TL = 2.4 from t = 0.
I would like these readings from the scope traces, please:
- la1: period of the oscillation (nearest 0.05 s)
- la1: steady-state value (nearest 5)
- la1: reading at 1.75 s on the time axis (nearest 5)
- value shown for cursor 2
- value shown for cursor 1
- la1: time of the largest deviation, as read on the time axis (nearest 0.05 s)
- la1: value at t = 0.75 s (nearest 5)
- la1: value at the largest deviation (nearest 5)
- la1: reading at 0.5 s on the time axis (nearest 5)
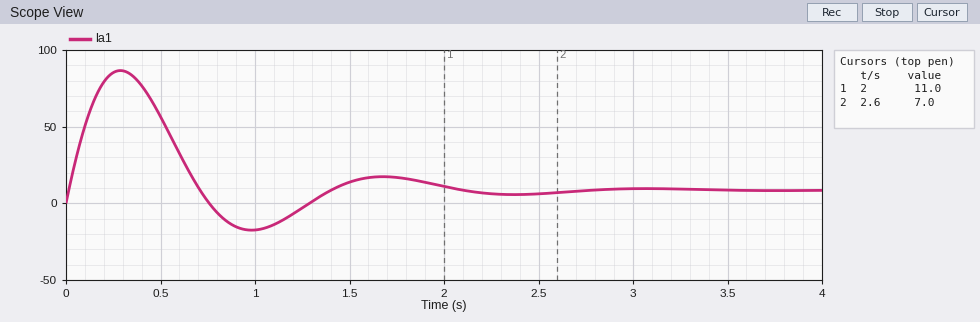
1.40 s
10
15
7.0
11.0
0.30 s
0
85
55
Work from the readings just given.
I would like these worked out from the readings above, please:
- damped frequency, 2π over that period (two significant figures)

4.5 rad/s
